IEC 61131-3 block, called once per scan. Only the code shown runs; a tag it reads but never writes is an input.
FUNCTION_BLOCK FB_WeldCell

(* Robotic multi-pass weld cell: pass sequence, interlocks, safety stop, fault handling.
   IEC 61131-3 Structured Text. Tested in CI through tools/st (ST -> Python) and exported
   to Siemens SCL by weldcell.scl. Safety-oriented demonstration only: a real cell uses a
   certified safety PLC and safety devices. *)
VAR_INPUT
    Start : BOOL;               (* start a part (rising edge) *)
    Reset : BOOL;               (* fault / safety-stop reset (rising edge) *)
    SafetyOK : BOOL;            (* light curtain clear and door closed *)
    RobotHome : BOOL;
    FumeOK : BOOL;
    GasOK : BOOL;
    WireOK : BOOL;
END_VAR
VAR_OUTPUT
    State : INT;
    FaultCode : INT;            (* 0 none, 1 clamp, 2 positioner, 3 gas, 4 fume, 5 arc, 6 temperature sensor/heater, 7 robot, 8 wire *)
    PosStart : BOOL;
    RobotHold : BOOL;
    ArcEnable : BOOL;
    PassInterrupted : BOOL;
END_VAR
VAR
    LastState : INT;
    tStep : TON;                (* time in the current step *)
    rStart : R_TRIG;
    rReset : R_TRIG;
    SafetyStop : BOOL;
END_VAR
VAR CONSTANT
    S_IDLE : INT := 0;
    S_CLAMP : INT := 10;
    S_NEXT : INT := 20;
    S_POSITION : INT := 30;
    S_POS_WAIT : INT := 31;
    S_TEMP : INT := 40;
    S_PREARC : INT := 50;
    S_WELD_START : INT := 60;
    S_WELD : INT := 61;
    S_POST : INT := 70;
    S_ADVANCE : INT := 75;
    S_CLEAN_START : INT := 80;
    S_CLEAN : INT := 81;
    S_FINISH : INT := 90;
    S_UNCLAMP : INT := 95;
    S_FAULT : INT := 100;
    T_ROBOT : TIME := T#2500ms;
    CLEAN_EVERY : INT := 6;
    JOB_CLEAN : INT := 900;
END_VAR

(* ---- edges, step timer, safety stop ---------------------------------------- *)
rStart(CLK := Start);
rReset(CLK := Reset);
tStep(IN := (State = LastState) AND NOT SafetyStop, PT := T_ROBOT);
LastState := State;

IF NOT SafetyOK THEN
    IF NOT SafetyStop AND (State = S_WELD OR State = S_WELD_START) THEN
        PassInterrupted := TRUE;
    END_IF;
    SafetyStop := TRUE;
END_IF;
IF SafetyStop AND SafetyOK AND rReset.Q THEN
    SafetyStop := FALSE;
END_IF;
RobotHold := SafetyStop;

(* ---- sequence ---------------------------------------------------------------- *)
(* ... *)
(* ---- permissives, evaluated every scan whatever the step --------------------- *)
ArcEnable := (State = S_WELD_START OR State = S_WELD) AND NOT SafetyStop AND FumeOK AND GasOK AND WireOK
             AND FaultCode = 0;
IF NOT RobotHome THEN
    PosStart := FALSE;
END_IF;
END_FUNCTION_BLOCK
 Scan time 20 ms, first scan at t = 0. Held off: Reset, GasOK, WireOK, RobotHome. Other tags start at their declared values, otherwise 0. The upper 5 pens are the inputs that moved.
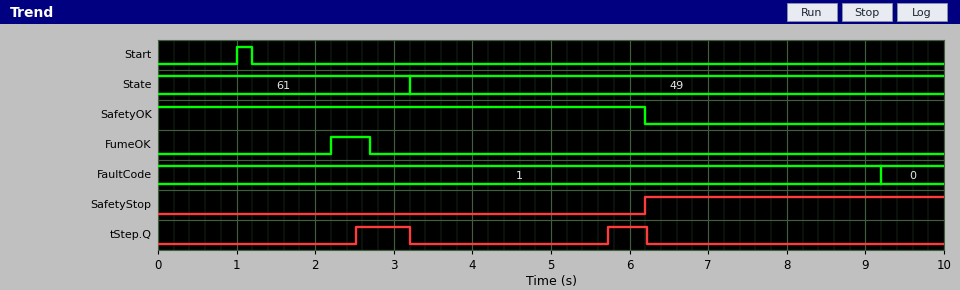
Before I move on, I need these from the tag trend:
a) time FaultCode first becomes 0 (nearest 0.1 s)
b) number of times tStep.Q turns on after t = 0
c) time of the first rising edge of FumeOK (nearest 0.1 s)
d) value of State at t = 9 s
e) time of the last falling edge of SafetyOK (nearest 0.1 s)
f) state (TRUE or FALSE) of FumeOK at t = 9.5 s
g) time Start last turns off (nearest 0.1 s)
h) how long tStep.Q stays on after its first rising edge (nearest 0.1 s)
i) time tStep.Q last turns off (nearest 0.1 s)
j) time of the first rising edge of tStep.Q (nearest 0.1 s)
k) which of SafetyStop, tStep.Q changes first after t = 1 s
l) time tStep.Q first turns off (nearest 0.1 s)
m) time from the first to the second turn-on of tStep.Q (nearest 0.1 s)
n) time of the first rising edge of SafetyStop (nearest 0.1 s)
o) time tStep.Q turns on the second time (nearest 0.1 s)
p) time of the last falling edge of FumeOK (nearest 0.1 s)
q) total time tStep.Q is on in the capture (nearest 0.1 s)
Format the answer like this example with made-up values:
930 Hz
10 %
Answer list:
9.2 s
2
2.2 s
49
6.2 s
FALSE
1.2 s
0.7 s
6.2 s
2.5 s
tStep.Q
3.2 s
3.2 s
6.2 s
5.7 s
2.7 s
1.2 s
